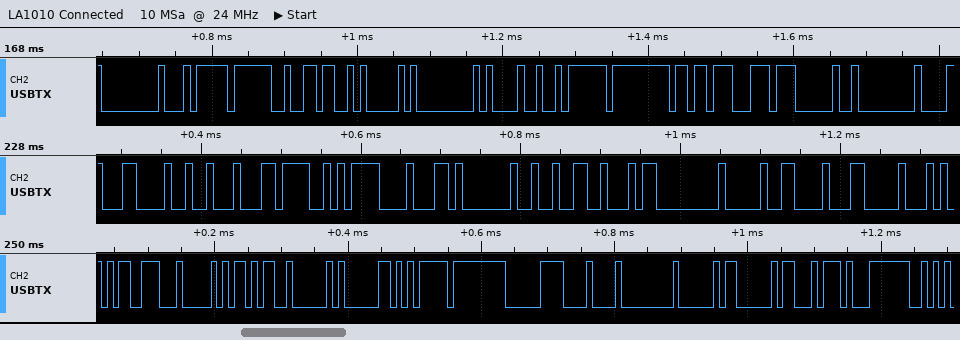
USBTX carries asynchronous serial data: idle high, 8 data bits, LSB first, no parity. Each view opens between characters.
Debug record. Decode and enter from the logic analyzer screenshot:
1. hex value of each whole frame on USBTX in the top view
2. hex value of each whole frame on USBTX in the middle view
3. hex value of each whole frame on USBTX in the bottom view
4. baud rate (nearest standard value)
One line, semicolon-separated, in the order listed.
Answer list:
00, F4, 3F, 36, 41, 00, 21, FA, FF, DB, DC, 20, 00; 0C, 12, EC, EA, 88, 01, 92, A2, 00, 90, 88, 10; CD, 04, AD, 02, 81, F5, FF, E0, 08, 00, A0, A0, 74, FC; 115200 baud
